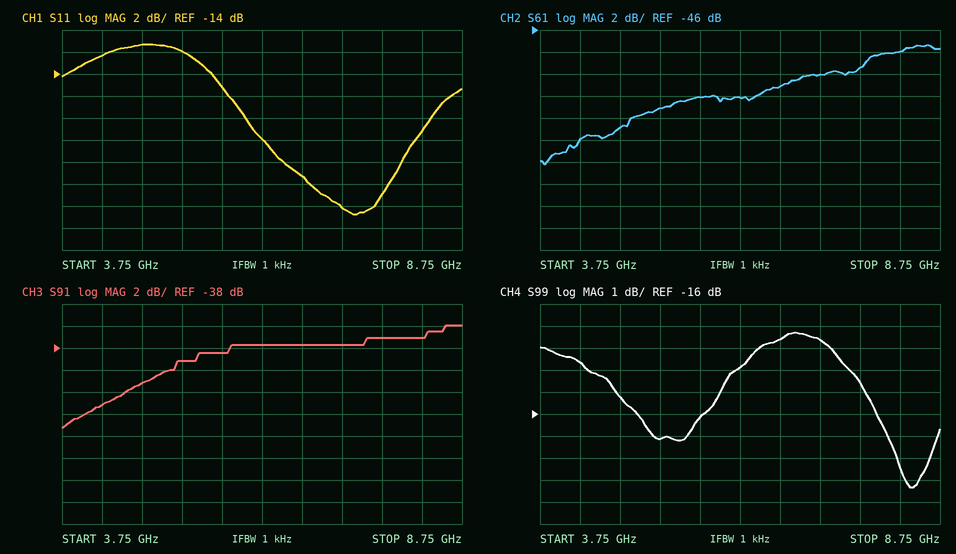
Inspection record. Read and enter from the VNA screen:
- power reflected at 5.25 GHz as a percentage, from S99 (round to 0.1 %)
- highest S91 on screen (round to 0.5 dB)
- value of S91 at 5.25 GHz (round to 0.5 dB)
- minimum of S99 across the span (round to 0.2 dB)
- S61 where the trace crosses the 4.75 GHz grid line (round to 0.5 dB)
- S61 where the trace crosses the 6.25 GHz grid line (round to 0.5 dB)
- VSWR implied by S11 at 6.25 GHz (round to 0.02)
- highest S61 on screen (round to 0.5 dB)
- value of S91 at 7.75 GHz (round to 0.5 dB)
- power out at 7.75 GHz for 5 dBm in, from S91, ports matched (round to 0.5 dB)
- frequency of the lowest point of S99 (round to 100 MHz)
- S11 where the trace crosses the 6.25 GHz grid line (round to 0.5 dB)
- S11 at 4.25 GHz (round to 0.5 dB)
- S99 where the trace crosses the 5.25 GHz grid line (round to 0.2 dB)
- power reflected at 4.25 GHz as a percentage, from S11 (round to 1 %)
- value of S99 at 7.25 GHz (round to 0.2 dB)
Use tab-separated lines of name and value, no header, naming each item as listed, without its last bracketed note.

power reflected at 5.25 GHz as a percentage, from S99	1.9 %
highest S91 on screen	-36.0 dB
value of S91 at 5.25 GHz	-39.0 dB
minimum of S99 across the span	-19.4 dB
S61 where the trace crosses the 4.75 GHz grid line	-55.0 dB
S61 where the trace crosses the 6.25 GHz grid line	-52.0 dB
VSWR implied by S11 at 6.25 GHz	1.22
highest S61 on screen	-47.5 dB
value of S91 at 7.75 GHz	-37.0 dB
power out at 7.75 GHz for 5 dBm in, from S91, ports matched	-32.0 dBm
frequency of the lowest point of S99	8.4 GHz
S11 where the trace crosses the 6.25 GHz grid line	-20.0 dB
S11 at 4.25 GHz	-12.5 dB
S99 where the trace crosses the 5.25 GHz grid line	-17.2 dB
power reflected at 4.25 GHz as a percentage, from S11	6 %
value of S99 at 7.25 GHz	-12.6 dB
